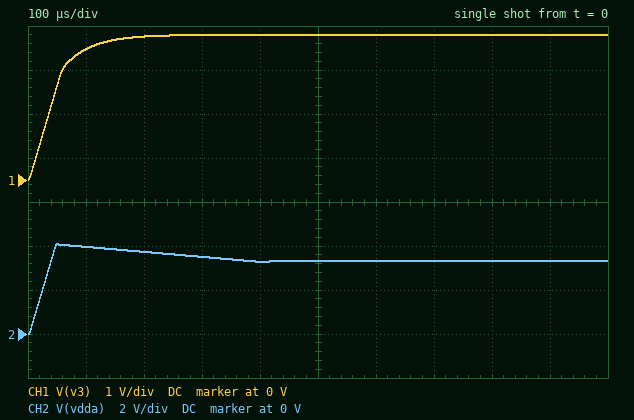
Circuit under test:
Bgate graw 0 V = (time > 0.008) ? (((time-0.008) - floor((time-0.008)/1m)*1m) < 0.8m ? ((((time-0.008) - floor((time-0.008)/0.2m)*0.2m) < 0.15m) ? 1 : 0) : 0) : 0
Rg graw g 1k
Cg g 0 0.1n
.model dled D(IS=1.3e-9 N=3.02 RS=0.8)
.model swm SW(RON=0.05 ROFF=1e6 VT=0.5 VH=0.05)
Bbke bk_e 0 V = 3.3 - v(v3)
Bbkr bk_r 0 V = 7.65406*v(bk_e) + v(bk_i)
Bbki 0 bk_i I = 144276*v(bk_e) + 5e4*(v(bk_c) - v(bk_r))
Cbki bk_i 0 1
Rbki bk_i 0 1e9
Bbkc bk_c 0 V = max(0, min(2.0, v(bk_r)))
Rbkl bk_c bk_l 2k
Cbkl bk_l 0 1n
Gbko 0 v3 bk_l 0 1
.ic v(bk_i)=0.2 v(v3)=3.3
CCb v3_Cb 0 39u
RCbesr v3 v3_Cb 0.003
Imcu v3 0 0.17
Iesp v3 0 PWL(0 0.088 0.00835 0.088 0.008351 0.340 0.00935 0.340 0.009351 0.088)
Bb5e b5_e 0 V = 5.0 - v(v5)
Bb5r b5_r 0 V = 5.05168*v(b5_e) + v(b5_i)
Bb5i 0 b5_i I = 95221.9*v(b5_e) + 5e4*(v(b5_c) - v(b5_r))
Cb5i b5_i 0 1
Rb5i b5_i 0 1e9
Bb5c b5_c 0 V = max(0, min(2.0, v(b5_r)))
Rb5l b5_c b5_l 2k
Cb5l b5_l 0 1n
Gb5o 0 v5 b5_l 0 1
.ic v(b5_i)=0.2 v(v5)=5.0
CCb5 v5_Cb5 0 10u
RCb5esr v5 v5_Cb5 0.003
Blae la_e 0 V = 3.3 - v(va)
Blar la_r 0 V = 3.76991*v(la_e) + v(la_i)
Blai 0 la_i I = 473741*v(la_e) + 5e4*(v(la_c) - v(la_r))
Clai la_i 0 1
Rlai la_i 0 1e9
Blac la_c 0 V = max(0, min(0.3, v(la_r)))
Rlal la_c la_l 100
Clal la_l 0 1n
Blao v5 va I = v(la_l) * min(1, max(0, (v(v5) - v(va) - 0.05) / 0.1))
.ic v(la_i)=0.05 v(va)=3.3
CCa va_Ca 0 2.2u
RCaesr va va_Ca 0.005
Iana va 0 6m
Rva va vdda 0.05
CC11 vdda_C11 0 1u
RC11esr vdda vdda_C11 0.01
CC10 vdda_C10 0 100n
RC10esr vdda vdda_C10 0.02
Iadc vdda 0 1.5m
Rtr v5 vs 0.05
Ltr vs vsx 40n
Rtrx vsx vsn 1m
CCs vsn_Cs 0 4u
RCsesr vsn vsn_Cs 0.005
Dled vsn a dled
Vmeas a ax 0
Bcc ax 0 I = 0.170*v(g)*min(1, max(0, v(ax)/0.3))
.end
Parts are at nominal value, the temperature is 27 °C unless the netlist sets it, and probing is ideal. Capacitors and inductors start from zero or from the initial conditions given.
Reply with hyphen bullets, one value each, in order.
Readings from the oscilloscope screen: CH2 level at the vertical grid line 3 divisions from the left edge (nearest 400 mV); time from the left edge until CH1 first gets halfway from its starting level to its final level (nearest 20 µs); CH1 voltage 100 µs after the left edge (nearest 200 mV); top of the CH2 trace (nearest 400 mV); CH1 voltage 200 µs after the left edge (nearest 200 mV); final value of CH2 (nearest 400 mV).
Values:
- 3.6 V
- 40 µs
- 3.0 V
- 4.0 V
- 3.2 V
- 3.2 V
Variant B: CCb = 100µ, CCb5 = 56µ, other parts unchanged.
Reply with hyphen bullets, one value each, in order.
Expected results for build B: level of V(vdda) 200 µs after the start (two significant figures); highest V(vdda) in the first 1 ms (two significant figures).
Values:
- 3.5 V
- 3.7 V
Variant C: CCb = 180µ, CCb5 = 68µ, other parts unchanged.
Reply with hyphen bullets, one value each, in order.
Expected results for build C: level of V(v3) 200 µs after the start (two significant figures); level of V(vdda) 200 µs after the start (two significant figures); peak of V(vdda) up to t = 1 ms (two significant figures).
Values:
- 1.9 V
- 3.5 V
- 3.6 V
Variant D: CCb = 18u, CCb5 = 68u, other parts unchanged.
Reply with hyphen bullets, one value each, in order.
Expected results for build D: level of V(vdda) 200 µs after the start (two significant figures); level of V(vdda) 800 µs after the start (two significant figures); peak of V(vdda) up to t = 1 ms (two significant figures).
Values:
- 3.5 V
- 3.3 V
- 3.6 V
